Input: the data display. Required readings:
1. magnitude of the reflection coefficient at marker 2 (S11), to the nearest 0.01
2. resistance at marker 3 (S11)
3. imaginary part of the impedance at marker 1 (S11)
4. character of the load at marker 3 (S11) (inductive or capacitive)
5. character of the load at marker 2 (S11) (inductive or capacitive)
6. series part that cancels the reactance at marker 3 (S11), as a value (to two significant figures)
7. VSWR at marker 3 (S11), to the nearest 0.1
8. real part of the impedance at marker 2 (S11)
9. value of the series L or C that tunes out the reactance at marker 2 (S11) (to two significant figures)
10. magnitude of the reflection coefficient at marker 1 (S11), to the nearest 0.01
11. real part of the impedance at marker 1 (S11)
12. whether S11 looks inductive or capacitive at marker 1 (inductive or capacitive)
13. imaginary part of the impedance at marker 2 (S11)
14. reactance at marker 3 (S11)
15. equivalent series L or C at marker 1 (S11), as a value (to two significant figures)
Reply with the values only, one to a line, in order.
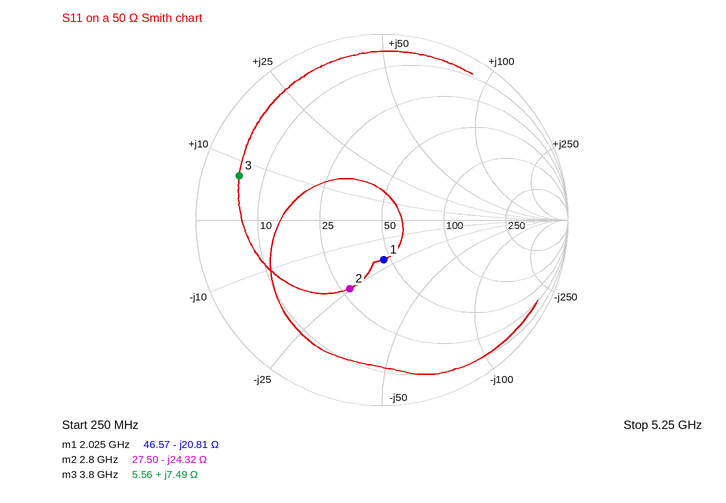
0.41
5.56 Ω
-20.81 Ω
inductive
capacitive
5.6 pF
9.2
27.50 Ω
1.4 nH
0.21
46.57 Ω
capacitive
-24.32 Ω
+7.49 Ω
3.8 pF
